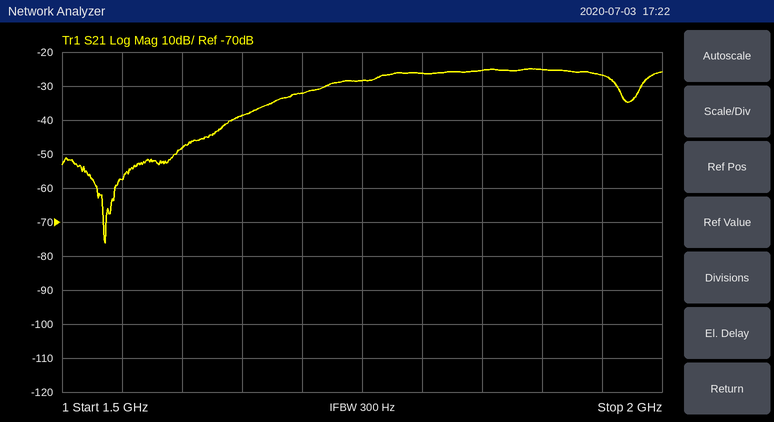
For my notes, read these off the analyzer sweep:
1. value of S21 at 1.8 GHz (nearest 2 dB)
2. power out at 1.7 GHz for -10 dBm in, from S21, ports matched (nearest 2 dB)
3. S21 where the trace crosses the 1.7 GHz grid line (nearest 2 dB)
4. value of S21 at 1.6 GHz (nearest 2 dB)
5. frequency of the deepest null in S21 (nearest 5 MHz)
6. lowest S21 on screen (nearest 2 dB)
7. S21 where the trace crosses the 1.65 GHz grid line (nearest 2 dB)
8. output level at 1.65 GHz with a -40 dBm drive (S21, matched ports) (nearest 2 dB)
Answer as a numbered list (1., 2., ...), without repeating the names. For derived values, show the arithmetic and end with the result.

1. -26 dB
2. -10 dBm + (-32 dB) = -42 dBm
3. -32 dB
4. -48 dB
5. 1.535 GHz
6. -76 dB
7. -38 dB
8. -40 dBm + (-38 dB) = -78 dBm
